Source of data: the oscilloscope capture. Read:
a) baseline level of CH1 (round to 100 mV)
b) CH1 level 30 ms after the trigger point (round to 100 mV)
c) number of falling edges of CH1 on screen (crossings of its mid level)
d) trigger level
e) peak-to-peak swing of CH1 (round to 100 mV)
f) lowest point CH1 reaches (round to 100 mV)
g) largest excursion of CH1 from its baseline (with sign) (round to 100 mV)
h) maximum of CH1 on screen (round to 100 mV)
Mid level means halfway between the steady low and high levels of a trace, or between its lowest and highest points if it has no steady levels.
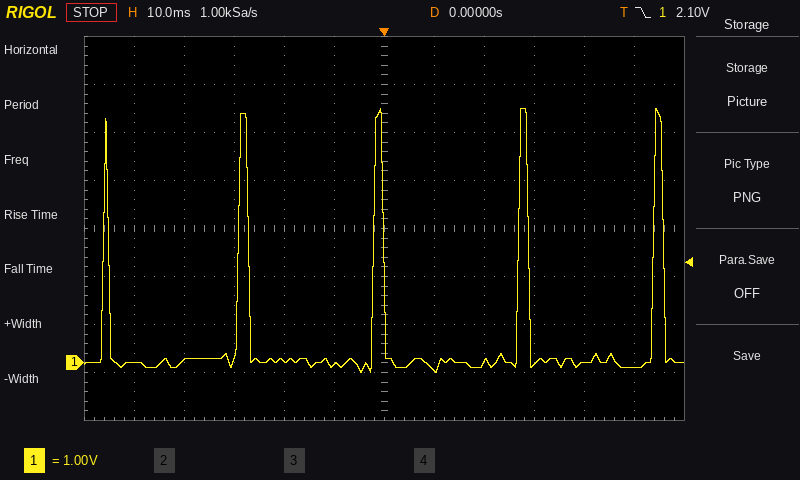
0.0 V
0.0 V
5
2.10 V
5.5 V
-200 mV
+5.3 V
5.3 V
